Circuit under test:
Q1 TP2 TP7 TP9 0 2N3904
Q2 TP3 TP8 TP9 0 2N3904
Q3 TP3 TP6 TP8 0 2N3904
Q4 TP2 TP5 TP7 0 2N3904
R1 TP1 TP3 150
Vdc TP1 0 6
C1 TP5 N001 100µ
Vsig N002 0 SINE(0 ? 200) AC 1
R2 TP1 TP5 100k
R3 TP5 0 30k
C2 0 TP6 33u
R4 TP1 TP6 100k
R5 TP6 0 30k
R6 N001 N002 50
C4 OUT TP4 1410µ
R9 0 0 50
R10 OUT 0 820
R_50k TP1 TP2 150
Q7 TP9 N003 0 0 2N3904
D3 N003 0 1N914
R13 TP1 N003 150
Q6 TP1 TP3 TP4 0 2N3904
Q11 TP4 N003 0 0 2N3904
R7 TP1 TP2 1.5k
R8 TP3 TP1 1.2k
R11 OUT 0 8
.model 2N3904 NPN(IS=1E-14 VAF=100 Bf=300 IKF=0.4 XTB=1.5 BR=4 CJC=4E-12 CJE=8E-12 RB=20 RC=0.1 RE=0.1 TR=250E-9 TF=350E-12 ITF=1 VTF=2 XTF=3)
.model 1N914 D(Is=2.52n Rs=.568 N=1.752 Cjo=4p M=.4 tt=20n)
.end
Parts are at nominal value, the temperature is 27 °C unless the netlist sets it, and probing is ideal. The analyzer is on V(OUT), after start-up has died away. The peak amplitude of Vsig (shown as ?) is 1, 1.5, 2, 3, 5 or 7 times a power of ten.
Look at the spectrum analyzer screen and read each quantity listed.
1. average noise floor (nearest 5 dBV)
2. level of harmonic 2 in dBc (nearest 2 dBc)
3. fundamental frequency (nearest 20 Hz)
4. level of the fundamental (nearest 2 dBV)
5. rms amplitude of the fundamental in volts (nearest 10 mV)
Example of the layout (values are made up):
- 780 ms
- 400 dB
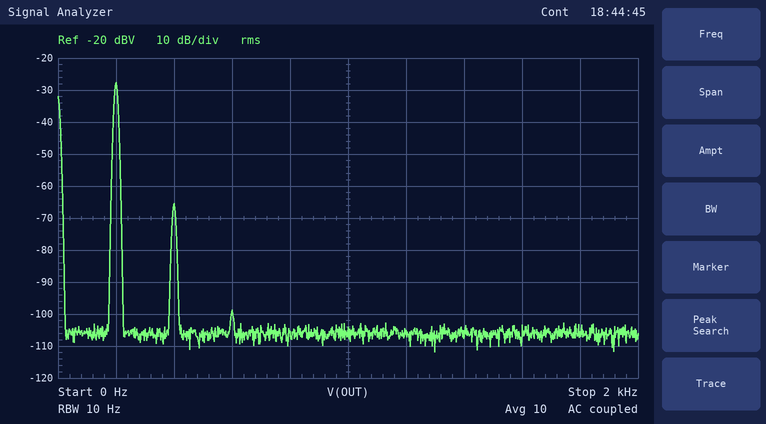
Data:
- -105 dBV
- -38 dBc
- 200 Hz
- -28 dBV
- 40 mV
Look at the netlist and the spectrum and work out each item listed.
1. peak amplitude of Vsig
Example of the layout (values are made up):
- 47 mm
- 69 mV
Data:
- 7 mV
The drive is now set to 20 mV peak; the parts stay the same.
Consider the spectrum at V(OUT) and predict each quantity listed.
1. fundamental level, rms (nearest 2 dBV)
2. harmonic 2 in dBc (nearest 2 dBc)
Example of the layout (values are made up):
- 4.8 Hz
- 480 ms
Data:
- -18 dBV
- -28 dBc
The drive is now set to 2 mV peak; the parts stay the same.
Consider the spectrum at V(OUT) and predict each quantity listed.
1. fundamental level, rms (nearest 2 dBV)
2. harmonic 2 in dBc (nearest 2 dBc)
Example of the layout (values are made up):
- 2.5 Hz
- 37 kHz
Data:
- -38 dBV
- -48 dBc
